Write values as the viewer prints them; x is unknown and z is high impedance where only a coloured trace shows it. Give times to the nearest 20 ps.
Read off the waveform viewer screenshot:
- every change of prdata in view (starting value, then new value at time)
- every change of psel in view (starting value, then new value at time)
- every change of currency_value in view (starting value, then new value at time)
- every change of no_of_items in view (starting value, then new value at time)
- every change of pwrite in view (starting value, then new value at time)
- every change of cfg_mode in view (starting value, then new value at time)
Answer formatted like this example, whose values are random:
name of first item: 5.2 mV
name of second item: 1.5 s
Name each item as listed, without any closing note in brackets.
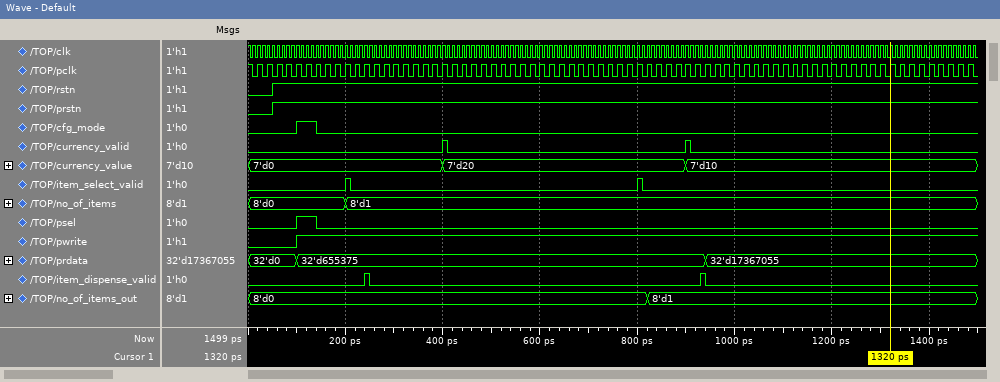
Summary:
every change of prdata in view: 32'd0, 32'd655375 at 100 ps, 32'd17367055 at 940 ps
every change of psel in view: 0, 1 at 100 ps, 0 at 140 ps
every change of currency_value in view: 7'd0, 7'd20 at 400 ps, 7'd10 at 900 ps
every change of no_of_items in view: 8'd0, 8'd1 at 200 ps
every change of pwrite in view: 0, 1 at 100 ps
every change of cfg_mode in view: 0, 1 at 100 ps, 0 at 140 ps
